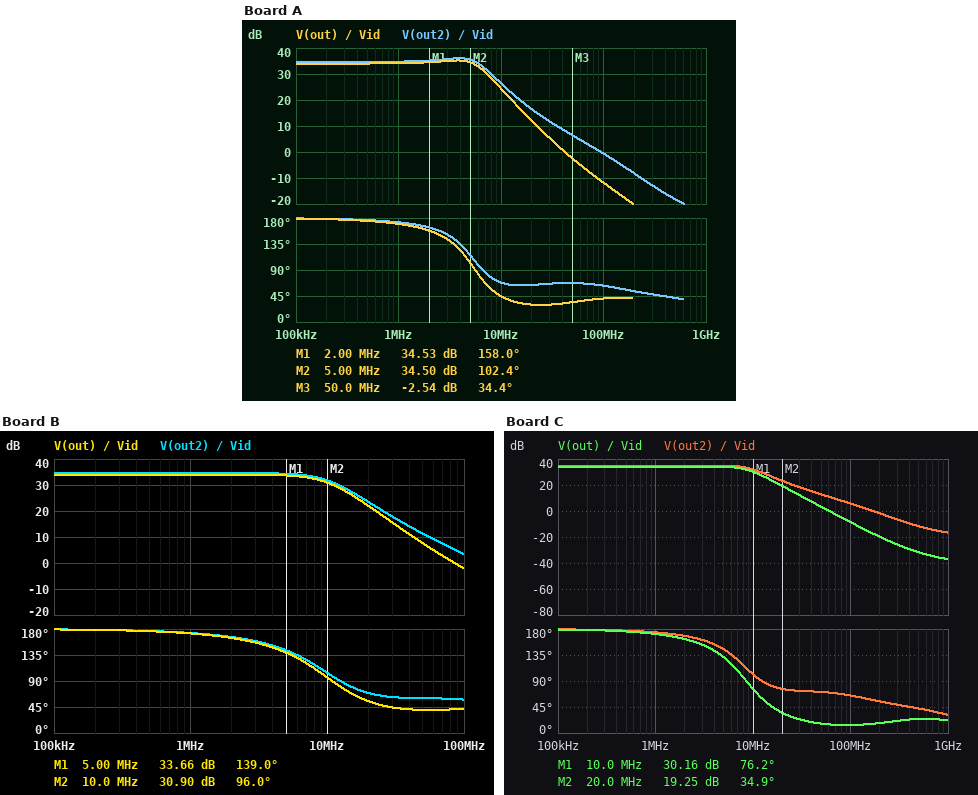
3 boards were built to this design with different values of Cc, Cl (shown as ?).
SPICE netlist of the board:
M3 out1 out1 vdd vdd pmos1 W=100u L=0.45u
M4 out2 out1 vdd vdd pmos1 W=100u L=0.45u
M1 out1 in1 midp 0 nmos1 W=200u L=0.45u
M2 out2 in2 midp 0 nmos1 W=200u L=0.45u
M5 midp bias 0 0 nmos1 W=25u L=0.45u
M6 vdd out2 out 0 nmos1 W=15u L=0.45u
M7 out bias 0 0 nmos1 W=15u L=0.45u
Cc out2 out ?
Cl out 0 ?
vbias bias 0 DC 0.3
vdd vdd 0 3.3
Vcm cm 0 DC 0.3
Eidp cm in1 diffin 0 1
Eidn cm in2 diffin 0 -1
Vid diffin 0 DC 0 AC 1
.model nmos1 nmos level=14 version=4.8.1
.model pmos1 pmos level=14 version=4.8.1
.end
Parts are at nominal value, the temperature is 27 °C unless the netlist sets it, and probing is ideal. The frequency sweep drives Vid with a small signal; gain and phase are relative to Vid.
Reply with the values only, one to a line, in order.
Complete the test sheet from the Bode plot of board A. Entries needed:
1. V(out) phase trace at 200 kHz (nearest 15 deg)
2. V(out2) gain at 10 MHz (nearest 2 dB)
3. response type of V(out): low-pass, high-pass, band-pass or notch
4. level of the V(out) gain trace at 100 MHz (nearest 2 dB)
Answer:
180 deg
26 dB
low-pass
-12 dB
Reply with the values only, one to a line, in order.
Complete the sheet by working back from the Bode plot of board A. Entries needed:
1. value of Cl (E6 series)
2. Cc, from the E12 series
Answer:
15 pF
4.7 pF
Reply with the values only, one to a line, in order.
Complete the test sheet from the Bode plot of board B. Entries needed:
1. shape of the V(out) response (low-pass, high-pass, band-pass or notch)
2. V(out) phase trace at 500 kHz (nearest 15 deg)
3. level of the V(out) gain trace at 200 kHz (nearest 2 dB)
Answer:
low-pass
180 deg
34 dB
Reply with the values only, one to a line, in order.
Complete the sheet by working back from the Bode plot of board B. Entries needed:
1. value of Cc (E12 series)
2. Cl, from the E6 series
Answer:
3.9 pF
4.7 pF
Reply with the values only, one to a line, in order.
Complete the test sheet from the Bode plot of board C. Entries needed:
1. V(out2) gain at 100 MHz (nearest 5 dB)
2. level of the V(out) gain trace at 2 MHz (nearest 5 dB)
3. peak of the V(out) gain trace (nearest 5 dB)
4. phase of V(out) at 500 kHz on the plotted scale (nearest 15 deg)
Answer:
5 dB
35 dB
35 dB
180 deg
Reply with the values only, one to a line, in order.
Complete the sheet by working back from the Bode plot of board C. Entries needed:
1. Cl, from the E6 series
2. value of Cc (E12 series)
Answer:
15 pF
1.5 pF
